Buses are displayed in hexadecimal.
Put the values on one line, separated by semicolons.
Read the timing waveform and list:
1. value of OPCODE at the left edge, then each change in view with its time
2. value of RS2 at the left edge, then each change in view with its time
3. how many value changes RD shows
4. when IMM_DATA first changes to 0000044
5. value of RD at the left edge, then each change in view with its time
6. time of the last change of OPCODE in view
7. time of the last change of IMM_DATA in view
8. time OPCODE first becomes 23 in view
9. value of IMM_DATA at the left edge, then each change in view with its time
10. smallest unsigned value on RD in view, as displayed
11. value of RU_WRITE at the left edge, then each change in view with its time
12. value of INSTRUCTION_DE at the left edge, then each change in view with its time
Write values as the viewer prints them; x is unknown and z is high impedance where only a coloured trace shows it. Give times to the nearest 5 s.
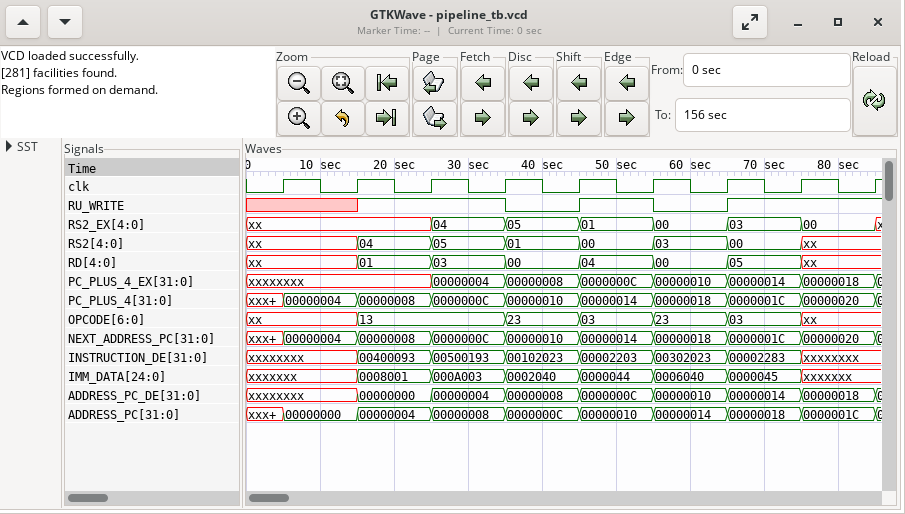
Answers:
xx, 13 at 15 s, 23 at 35 s, 03 at 45 s, 23 at 55 s, 03 at 65 s, xx at 75 s; xx, 04 at 15 s, 05 at 25 s, 01 at 35 s, 00 at 45 s, 03 at 55 s, 00 at 65 s, xx at 75 s; 7; 45 s; xx, 01 at 15 s, 03 at 25 s, 00 at 35 s, 04 at 45 s, 00 at 55 s, 05 at 65 s, xx at 75 s; 75 s; 75 s; 35 s; xxxxxxx, 0008001 at 15 s, 000A003 at 25 s, 0002040 at 35 s, 0000044 at 45 s, 0006040 at 55 s, 0000045 at 65 s, xxxxxxx at 75 s; 00; x, 1 at 15 s, 0 at 35 s, 1 at 45 s, 0 at 55 s, 1 at 65 s; xxxxxxxx, 00400093 at 15 s, 00500193 at 25 s, 00102023 at 35 s, 00002203 at 45 s, 00302023 at 55 s, 00002283 at 65 s, xxxxxxxx at 75 s
